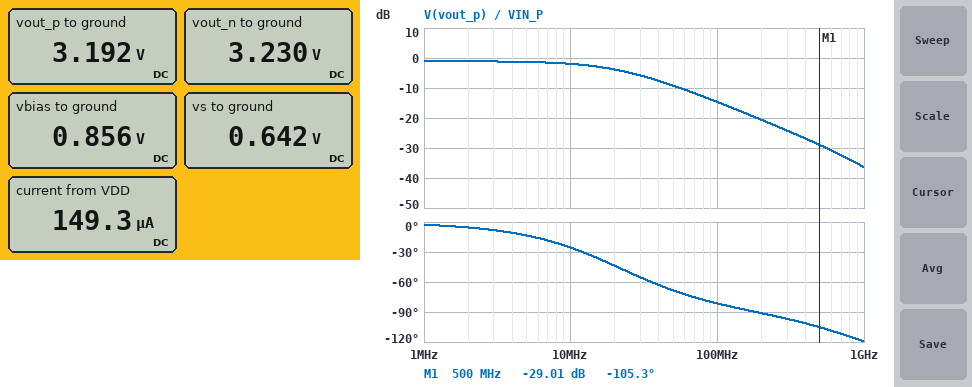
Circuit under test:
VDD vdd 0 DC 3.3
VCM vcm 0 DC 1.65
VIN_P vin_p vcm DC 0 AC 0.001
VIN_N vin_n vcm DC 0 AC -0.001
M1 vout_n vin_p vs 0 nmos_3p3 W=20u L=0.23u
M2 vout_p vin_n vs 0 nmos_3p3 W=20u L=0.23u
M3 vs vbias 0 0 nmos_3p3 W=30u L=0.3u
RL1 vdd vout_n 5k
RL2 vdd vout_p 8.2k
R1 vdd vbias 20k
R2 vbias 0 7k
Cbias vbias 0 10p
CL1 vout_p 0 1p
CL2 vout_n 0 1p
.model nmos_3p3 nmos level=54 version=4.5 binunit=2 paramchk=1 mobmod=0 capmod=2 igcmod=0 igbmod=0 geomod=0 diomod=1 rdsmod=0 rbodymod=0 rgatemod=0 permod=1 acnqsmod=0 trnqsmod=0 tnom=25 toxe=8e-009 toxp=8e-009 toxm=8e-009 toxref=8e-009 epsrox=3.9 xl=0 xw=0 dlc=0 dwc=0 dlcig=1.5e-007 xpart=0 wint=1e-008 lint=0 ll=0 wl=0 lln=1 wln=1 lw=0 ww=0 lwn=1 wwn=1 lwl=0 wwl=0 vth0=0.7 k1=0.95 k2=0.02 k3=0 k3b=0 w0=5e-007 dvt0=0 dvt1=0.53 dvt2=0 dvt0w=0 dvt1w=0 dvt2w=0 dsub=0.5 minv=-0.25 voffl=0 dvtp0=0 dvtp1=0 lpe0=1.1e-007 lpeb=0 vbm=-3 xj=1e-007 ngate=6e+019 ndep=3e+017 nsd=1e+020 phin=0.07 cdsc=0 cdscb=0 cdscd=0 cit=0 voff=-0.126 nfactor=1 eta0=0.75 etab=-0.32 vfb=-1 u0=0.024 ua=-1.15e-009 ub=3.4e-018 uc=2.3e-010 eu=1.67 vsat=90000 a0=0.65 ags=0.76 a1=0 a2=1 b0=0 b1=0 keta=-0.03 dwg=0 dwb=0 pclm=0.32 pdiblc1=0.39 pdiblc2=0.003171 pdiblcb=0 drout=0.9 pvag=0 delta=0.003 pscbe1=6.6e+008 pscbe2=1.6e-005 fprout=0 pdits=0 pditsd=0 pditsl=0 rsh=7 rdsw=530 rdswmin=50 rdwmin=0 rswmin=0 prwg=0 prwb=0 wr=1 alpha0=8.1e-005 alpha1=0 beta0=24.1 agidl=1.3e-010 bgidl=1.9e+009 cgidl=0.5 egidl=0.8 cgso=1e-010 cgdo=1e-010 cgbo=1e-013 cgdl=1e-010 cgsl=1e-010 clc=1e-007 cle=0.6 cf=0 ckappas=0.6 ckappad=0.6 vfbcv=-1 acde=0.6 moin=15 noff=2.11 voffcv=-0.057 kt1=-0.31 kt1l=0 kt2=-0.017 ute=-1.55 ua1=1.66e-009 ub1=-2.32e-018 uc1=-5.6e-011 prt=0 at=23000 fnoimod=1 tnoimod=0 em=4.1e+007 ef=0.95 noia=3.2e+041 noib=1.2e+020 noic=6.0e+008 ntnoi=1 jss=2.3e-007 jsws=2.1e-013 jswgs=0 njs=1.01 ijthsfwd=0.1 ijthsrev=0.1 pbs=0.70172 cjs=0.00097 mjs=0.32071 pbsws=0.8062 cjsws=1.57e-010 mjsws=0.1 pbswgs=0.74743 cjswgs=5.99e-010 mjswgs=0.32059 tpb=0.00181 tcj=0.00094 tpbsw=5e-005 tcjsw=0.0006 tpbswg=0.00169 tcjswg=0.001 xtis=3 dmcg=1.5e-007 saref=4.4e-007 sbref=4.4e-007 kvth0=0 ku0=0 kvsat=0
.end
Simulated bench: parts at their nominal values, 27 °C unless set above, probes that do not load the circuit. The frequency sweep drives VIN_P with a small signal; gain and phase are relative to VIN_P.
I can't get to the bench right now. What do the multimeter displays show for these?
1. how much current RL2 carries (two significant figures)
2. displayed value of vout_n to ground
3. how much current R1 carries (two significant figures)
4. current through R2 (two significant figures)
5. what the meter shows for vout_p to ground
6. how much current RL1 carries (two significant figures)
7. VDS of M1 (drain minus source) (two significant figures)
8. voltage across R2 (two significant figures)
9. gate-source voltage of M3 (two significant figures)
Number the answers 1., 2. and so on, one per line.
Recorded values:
1. 13 µA
2. 3.230 V
3. 120 µA
4. 120 µA
5. 3.192 V
6. 14 µA
7. 2.6 V
8. 860 mV
9. 860 mV
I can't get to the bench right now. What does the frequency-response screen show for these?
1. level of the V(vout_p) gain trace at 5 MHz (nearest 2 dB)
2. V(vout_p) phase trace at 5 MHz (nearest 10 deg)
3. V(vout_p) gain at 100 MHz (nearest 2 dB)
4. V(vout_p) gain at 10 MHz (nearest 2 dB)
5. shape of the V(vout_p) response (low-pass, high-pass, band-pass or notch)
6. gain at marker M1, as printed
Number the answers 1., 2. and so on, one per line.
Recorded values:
1. -2 dB
2. -10 deg
3. -14 dB
4. -2 dB
5. low-pass
6. -29.01 dB
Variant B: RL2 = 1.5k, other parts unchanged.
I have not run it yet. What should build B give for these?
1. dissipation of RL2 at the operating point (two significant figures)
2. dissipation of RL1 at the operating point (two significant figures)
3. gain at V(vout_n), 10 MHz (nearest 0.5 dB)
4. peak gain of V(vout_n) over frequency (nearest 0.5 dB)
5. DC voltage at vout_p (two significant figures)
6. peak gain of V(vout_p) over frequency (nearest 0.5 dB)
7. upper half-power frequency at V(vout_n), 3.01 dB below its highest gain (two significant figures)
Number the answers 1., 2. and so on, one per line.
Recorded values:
1. 300 nW
2. 880 nW
3. -5.0 dB
4. -4.5 dB
5. 3.3 V
6. -15.0 dB
7. 33 MHz
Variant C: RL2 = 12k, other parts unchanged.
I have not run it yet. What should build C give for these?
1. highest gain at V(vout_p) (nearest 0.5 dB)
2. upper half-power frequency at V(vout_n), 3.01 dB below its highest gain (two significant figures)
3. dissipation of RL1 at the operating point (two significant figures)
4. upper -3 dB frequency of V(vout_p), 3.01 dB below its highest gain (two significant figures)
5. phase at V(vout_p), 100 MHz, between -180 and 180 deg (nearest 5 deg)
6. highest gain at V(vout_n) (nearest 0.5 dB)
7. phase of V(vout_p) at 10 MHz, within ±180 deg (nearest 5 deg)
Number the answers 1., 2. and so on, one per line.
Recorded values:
1. 2.0 dB
2. 38 MHz
3. 1.0 µW
4. 15 MHz
5. -85 deg
6. -5.5 dB
7. -35 deg
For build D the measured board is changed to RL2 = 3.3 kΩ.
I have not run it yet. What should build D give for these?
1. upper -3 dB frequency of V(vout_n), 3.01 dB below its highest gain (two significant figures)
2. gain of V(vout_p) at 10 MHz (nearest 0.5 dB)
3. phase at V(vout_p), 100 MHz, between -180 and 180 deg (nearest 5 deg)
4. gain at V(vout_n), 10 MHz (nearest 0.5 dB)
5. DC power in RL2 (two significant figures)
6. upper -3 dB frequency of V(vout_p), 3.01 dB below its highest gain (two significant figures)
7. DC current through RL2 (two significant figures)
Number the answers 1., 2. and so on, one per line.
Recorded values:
1. 34 MHz
2. -8.5 dB
3. -65 deg
4. -5.0 dB
5. 630 nW
6. 52 MHz
7. 14 µA
